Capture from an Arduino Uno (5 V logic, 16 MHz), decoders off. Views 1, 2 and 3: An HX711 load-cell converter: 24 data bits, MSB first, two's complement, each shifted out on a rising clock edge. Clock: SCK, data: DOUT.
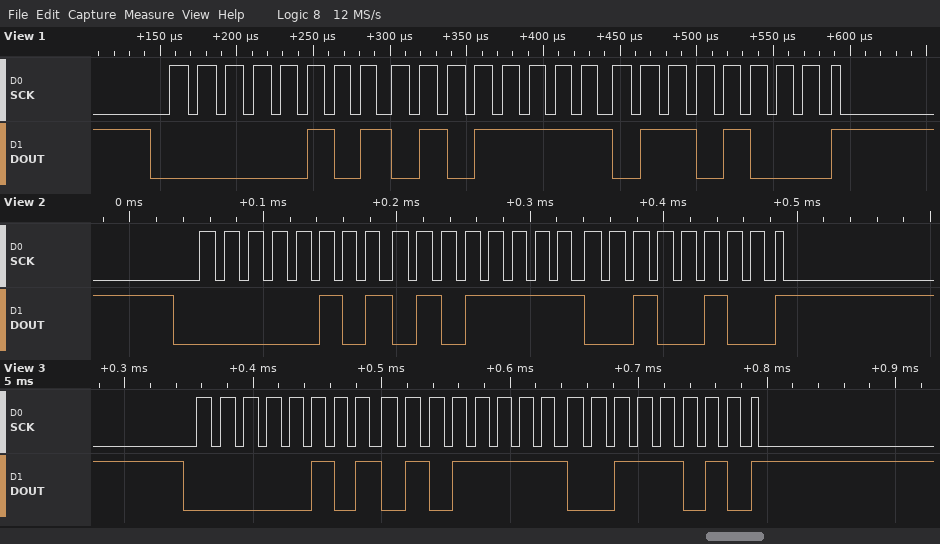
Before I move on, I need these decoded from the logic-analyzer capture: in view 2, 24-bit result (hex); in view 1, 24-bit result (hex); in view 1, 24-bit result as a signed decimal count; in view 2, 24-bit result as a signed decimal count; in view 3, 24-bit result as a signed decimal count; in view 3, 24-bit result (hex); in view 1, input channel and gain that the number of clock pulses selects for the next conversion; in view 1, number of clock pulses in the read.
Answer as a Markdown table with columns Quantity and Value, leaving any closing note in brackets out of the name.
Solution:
| Quantity | Value |
|---|---|
| in view 2, 24-bit result | 0x055F24 |
| in view 1, 24-bit result | 0x055F68 |
| in view 1, 24-bit result as a signed decimal count | 352104 |
| in view 2, 24-bit result as a signed decimal count | 352036 |
| in view 3, 24-bit result as a signed decimal count | 352058 |
| in view 3, 24-bit result | 0x055F3A |
| in view 1, input channel and gain that the number of clock pulses selects for the next conversion | channel A, gain 128 |
| in view 1, number of clock pulses in the read | 25 |
